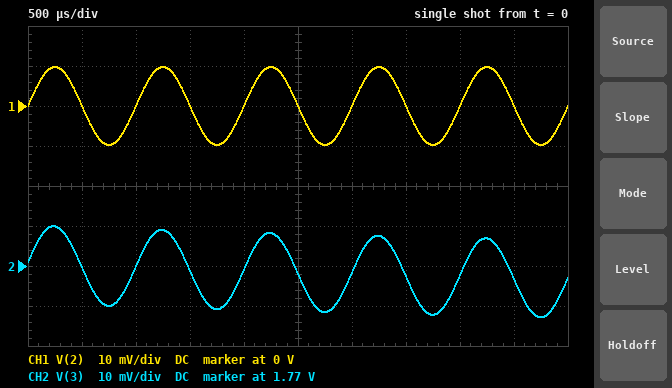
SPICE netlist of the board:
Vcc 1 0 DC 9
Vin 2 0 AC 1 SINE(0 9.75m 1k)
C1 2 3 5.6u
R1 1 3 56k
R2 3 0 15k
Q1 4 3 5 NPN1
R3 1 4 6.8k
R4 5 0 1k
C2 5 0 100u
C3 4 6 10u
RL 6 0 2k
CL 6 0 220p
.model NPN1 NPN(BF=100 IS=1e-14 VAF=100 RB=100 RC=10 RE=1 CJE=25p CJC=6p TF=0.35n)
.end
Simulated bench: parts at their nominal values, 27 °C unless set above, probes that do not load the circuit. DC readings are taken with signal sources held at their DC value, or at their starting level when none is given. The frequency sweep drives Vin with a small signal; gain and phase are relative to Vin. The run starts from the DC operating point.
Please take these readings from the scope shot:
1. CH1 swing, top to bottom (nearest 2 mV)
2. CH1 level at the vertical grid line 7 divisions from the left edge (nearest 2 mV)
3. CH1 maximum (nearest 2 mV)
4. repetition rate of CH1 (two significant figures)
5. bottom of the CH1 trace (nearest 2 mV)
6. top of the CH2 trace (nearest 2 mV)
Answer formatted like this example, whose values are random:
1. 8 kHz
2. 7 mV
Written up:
1. 20 mV
2. 0 V
3. 10 mV
4. 1.0 kHz
5. -10 mV
6. 1.780 V
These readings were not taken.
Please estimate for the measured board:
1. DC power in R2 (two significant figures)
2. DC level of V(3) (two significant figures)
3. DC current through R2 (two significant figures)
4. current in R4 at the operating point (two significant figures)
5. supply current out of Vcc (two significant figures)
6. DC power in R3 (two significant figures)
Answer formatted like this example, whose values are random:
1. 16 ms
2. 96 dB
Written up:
1. 210 µW
2. 1.8 V
3. 120 µA
4. 1.1 mA
5. 1.2 mA
6. 8.2 mW
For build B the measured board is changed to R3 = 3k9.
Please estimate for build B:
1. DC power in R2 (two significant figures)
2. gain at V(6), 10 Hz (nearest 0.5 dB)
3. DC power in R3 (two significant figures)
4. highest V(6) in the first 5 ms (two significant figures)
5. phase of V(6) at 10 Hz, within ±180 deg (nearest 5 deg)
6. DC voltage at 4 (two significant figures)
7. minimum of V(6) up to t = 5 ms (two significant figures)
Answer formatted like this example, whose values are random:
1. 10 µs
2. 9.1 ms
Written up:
1. 210 µW
2. 16.0 dB
3. 4.8 mW
4. 460 mV
5. -80 deg
6. 4.7 V
7. -530 mV
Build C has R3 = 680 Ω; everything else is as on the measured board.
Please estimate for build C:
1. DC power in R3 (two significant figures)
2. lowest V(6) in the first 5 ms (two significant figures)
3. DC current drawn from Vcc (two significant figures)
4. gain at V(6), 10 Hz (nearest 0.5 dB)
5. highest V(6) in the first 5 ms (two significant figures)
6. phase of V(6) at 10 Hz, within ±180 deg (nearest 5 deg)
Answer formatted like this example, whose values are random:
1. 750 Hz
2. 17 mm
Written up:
1. 840 µW
2. -210 mV
3. 1.2 mA
4. 7.0 dB
5. 180 mV
6. -65 deg
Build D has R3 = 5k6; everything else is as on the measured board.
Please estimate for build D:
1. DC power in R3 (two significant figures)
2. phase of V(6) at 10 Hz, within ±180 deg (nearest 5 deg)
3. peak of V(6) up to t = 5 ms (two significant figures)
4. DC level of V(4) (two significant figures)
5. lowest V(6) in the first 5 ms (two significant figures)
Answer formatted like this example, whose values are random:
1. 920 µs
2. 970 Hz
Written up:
1. 6.8 mW
2. -80 deg
3. 510 mV
4. 2.8 V
5. -590 mV
